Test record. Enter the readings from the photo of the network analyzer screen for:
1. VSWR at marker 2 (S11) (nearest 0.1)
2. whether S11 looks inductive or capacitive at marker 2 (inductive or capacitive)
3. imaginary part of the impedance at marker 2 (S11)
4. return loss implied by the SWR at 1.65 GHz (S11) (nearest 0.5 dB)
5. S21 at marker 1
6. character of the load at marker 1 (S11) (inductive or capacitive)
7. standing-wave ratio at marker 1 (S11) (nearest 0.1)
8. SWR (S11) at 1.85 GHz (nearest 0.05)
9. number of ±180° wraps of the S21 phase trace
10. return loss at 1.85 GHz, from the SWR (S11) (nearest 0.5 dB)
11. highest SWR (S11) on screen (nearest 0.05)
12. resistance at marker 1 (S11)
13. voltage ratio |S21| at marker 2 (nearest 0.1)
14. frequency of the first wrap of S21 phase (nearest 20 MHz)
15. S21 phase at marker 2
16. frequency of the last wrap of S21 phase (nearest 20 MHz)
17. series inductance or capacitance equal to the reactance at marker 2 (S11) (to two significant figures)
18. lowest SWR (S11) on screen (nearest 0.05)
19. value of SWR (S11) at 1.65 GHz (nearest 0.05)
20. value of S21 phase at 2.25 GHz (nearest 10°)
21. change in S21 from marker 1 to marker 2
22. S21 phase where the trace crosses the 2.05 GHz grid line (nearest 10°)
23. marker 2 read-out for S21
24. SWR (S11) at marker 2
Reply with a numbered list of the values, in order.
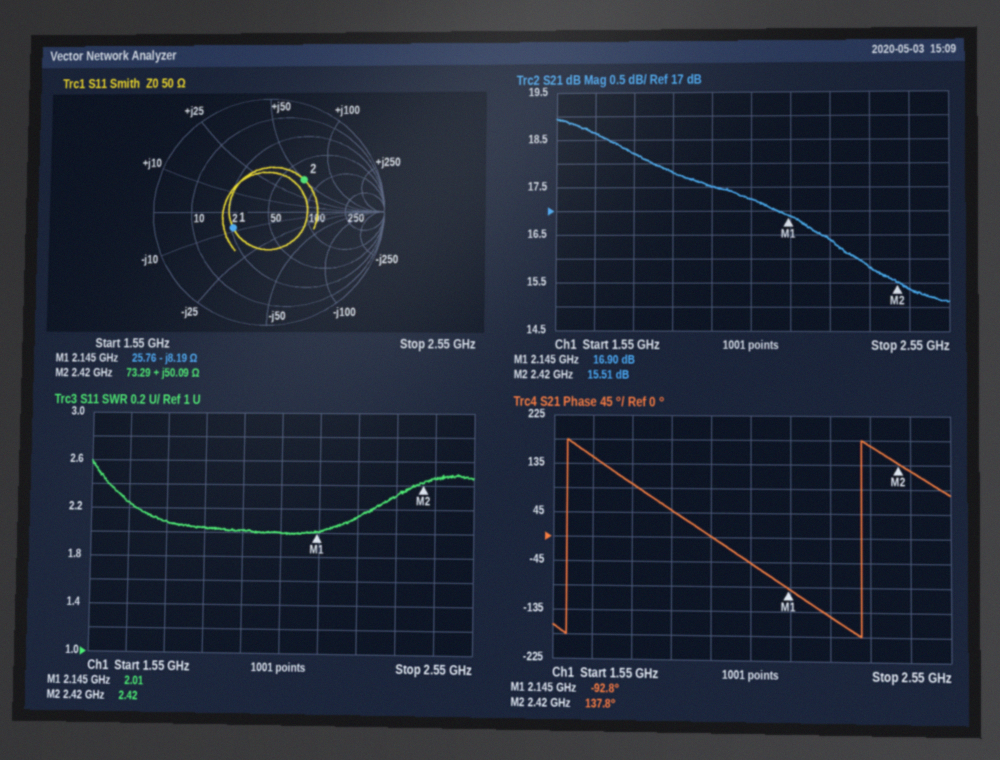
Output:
1. 2.4
2. inductive
3. +50.09 Ω
4. 8.5 dB
5. 16.90 dB
6. capacitive
7. 2.0
8. 2.05
9. 2
10. 9.5 dB
11. 2.60
12. 25.76 Ω
13. 6.0
14. 1.58 GHz
15. 137.8°
16. 2.32 GHz
17. 3.3 nH
18. 2.00
19. 2.25
20. -140°
21. -1.39 dB
22. -50°
23. 15.51 dB
24. 2.42
